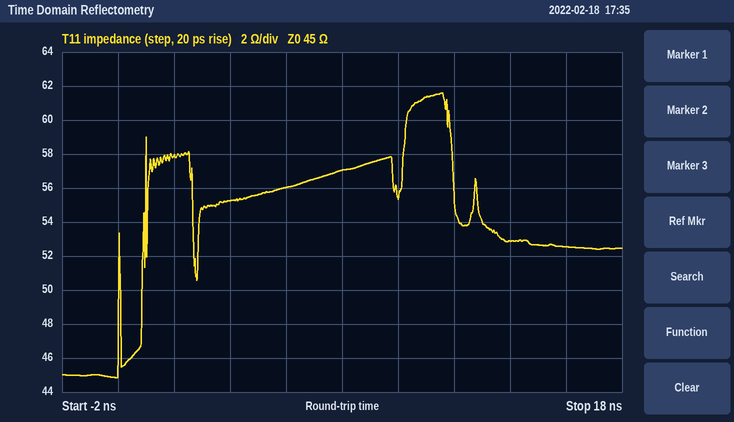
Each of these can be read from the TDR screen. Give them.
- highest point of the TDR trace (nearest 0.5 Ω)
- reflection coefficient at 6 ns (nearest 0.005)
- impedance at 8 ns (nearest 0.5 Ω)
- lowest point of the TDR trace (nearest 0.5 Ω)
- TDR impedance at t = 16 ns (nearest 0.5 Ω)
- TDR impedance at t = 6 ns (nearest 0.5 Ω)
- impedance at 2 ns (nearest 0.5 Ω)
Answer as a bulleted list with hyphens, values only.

- 61.5 Ω
- +0.110
- 57.0 Ω
- 45.0 Ω
- 52.5 Ω
- 56.0 Ω
- 58.0 Ω
